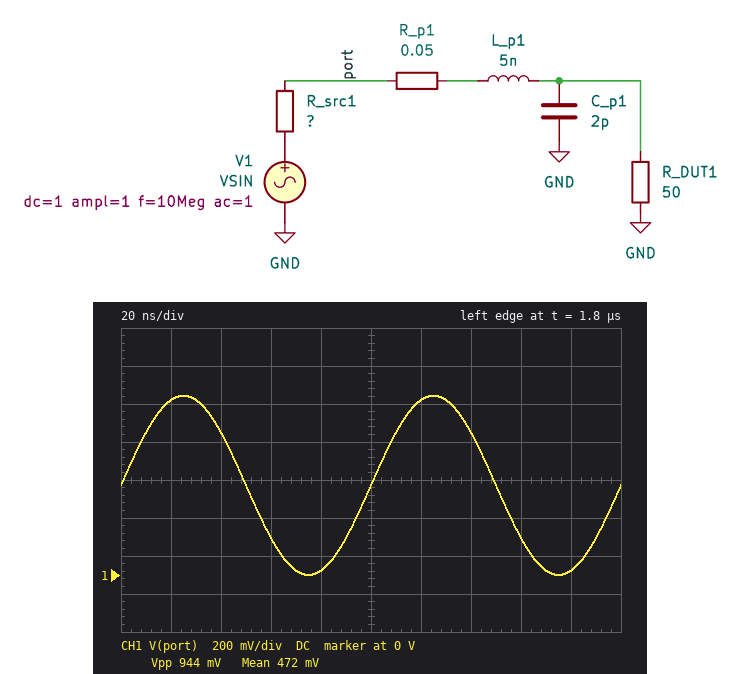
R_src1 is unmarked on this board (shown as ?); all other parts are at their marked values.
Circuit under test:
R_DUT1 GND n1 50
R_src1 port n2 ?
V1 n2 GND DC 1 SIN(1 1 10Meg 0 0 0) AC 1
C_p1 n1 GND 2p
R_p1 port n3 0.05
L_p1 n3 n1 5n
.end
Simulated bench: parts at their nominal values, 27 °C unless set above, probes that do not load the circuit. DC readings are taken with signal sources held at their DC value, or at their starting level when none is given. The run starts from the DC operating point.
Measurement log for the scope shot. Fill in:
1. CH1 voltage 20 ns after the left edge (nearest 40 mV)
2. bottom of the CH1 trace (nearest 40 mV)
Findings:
920 mV
0 V
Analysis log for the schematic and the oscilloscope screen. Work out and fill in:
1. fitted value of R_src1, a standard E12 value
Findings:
56 Ω
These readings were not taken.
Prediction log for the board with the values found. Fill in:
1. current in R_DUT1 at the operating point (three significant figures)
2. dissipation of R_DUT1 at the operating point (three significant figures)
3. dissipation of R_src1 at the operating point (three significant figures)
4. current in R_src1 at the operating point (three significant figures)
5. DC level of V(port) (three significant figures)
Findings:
9.43 mA
4.45 mW
4.98 mW
9.43 mA
472 mV
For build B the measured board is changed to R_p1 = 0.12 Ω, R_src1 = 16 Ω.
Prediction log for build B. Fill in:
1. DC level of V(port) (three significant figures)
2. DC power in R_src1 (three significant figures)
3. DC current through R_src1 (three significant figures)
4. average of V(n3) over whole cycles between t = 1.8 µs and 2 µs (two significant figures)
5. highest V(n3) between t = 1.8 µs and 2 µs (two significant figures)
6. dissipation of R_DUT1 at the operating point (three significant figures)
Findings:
758 mV
3.66 mW
15.1 mA
760 mV
1.5 V
11.4 mW
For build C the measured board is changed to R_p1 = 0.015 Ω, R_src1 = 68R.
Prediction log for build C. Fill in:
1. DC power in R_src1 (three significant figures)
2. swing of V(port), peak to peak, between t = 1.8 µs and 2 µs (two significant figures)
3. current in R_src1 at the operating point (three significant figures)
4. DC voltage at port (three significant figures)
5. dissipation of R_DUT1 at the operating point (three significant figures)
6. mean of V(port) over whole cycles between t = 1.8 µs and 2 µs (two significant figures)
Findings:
4.88 mW
850 mV
8.47 mA
424 mV
3.59 mW
420 mV
